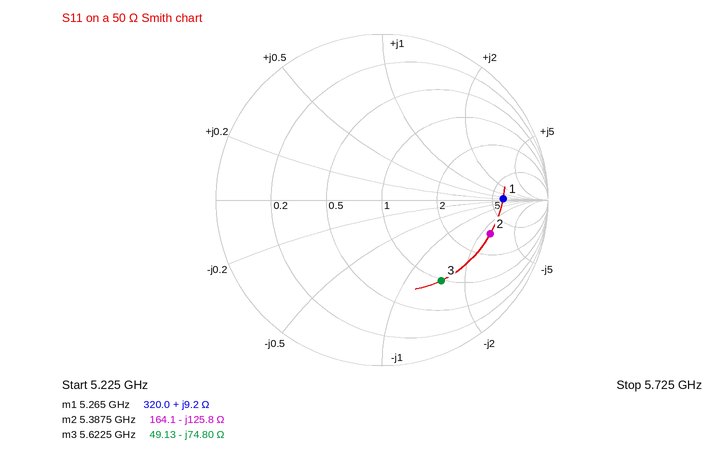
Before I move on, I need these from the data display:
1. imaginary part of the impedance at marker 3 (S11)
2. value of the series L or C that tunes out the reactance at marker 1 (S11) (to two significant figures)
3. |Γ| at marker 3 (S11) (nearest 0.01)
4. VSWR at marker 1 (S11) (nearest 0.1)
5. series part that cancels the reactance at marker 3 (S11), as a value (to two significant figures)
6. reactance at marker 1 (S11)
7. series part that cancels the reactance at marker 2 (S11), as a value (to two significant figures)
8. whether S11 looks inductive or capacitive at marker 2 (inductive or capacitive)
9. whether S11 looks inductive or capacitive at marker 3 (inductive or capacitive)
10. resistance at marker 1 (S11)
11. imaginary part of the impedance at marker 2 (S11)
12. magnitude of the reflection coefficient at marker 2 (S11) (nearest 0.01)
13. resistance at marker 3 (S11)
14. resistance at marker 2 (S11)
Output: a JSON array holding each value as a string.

["-74.80 Ω", "3.3 pF", "0.60", "6.4", "2.1 nH", "+9.2 Ω", "3.7 nH", "capacitive", "capacitive", "320.0 Ω", "-125.8 Ω", "0.68", "49.13 Ω", "164.1 Ω"]
